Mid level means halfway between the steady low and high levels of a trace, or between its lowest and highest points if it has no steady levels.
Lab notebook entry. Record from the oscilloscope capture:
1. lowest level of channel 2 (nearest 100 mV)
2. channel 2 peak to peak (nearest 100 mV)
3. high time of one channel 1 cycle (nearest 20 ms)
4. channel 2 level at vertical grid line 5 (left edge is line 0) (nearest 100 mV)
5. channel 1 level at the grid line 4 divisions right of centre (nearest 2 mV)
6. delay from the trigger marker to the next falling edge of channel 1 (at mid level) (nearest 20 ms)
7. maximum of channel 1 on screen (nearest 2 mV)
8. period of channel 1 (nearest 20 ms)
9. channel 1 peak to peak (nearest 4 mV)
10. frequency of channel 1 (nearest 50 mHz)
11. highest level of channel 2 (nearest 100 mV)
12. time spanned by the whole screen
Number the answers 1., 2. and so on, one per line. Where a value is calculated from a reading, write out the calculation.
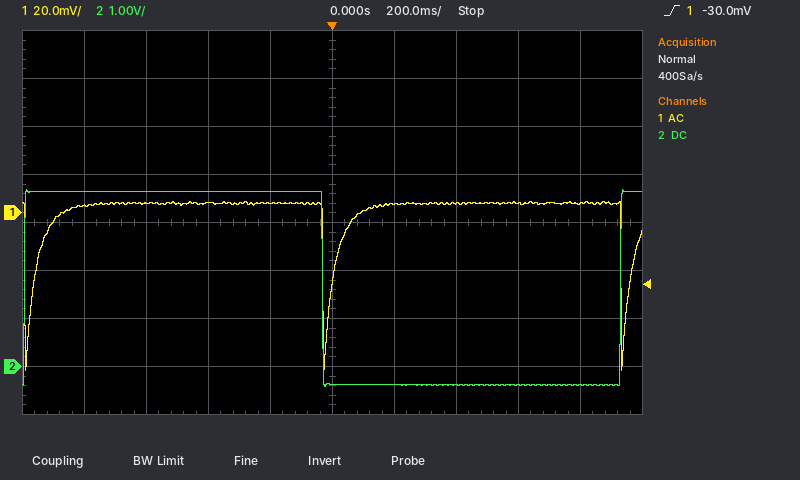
1. -400 mV
2. 3.7 V − (-400 mV) = 4.1 V
3. 940 ms
4. -400 mV
5. 4 mV
6. 940 ms
7. 4 mV
8. 960 ms
9. 72 mV
10. 1 / 960 ms ≈ 1.04 Hz, so 1.05 Hz to the nearest 50 mHz
11. 3.7 V
12. 2 s
